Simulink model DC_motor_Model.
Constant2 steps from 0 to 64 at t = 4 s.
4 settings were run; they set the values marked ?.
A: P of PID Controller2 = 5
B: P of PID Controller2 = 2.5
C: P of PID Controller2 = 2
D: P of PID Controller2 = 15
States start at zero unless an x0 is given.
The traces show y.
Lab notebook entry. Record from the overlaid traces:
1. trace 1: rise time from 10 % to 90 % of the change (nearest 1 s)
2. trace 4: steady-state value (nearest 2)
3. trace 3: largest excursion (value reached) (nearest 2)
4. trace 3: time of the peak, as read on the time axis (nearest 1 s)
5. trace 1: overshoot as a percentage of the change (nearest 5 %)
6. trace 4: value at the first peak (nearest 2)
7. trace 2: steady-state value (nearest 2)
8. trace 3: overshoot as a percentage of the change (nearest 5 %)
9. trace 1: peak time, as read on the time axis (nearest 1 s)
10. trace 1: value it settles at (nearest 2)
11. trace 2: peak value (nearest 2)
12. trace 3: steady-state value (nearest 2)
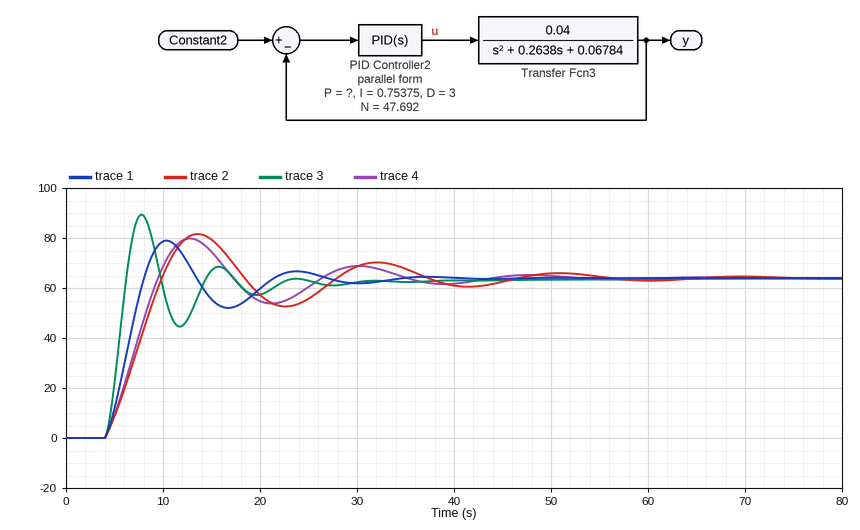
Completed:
3 s
64
90
8 s
25 %
80
64
40 %
10 s
64
82
64
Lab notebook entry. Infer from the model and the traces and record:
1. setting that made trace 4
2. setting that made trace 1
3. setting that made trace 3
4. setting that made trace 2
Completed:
B
A
D
C
